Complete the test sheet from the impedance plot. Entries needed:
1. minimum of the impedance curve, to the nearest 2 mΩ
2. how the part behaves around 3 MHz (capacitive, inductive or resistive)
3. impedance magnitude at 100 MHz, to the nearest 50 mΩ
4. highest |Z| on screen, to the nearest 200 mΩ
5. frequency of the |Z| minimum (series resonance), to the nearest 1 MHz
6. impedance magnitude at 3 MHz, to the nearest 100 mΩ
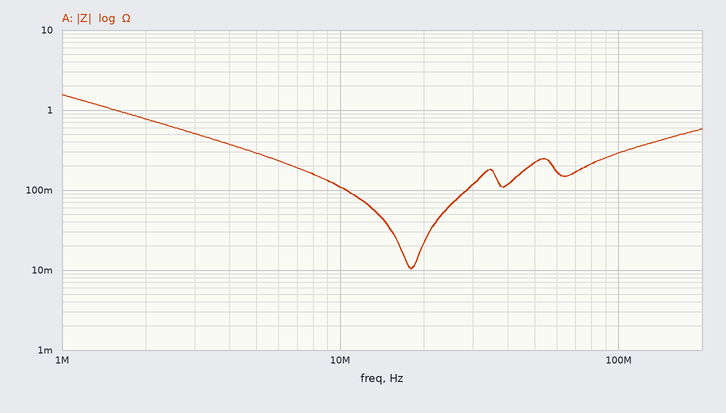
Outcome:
10 mΩ
capacitive
300 mΩ
1.6 Ω
18 MHz
500 mΩ
